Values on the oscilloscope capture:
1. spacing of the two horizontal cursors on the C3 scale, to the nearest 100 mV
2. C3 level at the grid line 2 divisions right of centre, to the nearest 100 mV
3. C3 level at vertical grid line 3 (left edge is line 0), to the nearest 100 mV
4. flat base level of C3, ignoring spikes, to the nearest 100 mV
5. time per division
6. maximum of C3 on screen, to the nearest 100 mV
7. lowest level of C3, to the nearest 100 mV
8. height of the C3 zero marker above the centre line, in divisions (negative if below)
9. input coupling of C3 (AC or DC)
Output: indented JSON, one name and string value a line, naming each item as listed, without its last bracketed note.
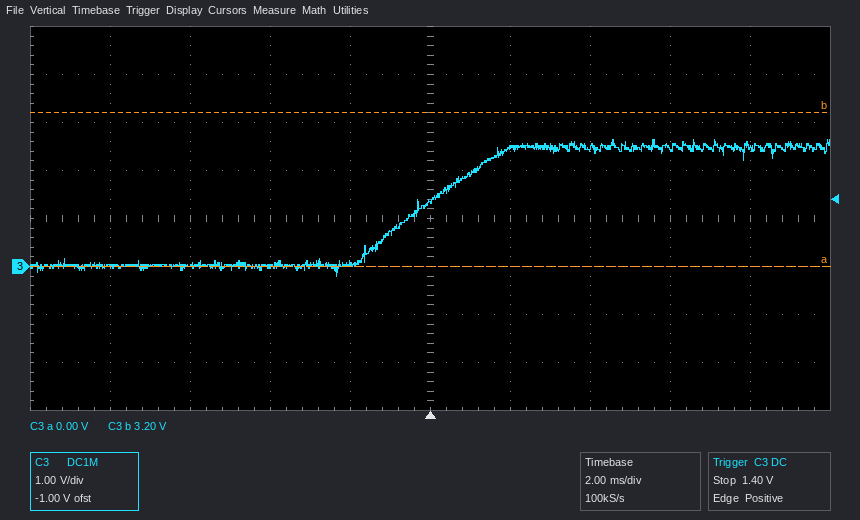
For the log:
{
  "spacing of the two horizontal cursors on the C3 scale, to the nearest 100 mV": "3.2 V",
  "C3 level at the grid line 2 divisions right of centre, to the nearest 100 mV": "2.5 V",
  "C3 level at vertical grid line 3 (left edge is line 0), to the nearest 100 mV": "0.0 V",
  "flat base level of C3, ignoring spikes, to the nearest 100 mV": "0.0 V",
  "time per division": "2 ms",
  "maximum of C3 on screen, to the nearest 100 mV": "2.6 V",
  "lowest level of C3, to the nearest 100 mV": "-200 mV",
  "height of the C3 zero marker above the centre line, in divisions": "-1.0 div",
  "input coupling of C3": "DC"
}
